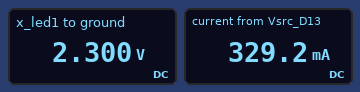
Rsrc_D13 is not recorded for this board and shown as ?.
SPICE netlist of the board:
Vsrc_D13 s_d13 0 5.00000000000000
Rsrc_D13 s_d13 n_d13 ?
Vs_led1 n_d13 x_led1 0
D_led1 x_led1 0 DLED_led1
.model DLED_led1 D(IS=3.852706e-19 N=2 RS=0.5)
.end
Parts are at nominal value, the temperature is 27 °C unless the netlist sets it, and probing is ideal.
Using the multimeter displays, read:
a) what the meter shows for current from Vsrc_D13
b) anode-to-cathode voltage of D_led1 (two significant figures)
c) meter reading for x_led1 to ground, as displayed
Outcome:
329.2 mA
2.3 V
2.300 V
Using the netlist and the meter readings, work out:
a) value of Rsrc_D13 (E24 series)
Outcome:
8.2 Ω
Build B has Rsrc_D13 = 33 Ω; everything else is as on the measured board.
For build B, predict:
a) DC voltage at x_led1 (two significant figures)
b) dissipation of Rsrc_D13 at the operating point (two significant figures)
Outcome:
2.1 V
250 mW
